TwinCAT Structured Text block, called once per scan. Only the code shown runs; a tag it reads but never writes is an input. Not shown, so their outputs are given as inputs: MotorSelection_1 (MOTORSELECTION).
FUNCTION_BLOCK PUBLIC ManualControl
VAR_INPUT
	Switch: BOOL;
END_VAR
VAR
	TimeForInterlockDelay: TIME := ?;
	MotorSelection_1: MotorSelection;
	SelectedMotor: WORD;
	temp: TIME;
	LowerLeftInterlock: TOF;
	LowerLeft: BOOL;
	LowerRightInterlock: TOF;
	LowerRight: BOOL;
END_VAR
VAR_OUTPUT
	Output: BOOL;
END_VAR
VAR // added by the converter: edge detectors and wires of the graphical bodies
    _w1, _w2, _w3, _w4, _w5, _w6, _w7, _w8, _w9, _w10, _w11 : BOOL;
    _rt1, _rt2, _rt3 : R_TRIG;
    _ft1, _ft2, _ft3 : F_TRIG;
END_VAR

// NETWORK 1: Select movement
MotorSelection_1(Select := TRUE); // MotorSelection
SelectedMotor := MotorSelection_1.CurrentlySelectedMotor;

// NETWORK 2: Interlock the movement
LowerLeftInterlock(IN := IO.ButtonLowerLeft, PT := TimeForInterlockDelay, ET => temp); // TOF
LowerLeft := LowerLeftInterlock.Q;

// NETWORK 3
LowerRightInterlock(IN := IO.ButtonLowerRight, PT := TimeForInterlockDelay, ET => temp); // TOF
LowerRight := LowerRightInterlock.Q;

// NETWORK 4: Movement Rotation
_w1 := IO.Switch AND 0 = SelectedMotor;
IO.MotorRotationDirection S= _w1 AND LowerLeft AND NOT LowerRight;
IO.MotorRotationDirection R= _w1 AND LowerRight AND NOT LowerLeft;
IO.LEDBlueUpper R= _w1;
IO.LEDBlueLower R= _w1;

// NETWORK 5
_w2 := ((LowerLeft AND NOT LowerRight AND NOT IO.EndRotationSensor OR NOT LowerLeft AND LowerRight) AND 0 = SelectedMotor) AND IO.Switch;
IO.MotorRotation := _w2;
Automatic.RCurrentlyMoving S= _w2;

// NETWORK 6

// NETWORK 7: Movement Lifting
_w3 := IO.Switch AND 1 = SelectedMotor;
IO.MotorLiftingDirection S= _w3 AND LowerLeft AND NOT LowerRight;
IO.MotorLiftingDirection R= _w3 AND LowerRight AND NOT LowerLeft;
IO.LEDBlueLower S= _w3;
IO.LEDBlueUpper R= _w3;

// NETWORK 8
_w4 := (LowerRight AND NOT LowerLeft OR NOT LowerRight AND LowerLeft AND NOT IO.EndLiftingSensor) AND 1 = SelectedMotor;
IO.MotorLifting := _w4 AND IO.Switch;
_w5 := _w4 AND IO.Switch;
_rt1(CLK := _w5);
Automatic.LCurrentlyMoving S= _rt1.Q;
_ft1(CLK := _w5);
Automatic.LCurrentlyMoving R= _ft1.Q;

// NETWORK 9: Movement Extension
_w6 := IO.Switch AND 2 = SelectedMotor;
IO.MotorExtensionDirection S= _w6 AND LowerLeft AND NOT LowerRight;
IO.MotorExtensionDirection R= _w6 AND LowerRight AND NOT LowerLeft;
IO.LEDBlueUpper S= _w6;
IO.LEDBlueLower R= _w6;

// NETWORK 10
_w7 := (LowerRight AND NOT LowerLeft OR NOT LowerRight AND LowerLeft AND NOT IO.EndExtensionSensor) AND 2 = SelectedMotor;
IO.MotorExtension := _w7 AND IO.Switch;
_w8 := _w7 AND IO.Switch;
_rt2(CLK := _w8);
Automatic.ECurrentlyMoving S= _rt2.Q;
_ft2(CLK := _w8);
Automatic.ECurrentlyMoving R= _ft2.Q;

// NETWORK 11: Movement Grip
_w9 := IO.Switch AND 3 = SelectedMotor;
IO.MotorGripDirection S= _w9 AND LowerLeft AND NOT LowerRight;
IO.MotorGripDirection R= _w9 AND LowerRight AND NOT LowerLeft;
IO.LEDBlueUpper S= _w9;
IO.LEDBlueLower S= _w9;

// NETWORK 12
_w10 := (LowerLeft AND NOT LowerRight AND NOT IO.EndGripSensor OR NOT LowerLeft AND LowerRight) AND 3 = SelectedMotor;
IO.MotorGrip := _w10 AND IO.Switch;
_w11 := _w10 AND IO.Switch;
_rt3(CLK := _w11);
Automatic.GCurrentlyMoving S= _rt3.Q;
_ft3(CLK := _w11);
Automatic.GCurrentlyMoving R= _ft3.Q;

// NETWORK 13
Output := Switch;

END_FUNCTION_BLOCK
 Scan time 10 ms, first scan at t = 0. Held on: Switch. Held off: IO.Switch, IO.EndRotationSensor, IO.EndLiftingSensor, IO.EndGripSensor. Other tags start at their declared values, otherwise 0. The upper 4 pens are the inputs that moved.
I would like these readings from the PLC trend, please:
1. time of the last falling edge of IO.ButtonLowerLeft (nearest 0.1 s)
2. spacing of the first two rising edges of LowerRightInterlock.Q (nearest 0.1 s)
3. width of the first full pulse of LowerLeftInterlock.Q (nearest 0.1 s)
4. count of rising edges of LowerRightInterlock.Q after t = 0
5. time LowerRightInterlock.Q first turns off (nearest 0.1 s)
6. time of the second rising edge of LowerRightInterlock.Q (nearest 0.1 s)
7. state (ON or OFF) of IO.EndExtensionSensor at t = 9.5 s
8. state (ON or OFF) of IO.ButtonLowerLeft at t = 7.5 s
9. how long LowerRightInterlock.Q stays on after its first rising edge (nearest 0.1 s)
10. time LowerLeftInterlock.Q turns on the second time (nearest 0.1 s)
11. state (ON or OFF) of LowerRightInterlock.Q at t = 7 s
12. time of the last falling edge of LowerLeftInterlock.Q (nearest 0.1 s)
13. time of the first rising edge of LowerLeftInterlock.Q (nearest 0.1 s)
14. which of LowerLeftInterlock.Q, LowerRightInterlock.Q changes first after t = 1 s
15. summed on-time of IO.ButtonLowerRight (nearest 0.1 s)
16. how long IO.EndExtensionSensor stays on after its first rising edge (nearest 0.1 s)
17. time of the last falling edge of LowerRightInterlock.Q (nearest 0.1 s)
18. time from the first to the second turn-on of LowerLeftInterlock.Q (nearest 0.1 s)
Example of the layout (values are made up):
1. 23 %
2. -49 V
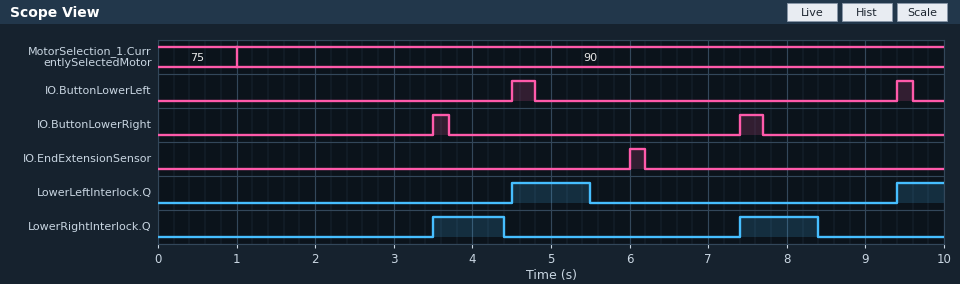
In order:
1. 9.6 s
2. 3.9 s
3. 1.0 s
4. 2
5. 4.4 s
6. 7.4 s
7. OFF
8. OFF
9. 0.9 s
10. 9.4 s
11. OFF
12. 5.5 s
13. 4.5 s
14. LowerRightInterlock.Q
15. 0.5 s
16. 0.2 s
17. 8.4 s
18. 4.9 s
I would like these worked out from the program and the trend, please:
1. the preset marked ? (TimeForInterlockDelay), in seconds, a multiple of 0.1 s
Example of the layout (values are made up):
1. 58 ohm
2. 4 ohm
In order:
1. 0.7 s
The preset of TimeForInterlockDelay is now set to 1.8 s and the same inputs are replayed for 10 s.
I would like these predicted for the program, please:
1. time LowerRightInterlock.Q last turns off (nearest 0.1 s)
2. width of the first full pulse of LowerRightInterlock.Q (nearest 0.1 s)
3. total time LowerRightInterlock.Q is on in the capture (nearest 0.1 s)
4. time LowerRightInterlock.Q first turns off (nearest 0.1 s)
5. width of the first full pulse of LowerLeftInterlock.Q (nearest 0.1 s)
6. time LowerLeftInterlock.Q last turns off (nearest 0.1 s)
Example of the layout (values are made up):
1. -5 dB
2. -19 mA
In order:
1. 9.5 s
2. 2.0 s
3. 4.1 s
4. 5.5 s
5. 2.1 s
6. 6.6 s
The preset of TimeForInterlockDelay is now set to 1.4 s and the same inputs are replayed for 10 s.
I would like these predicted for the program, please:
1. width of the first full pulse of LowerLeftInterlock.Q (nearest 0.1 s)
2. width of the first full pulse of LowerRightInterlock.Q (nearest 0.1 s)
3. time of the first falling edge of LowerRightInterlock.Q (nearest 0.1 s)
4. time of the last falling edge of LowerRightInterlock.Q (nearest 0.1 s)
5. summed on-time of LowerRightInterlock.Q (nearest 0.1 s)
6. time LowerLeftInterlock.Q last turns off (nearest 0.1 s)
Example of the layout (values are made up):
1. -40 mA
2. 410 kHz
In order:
1. 1.7 s
2. 1.6 s
3. 5.1 s
4. 9.1 s
5. 3.3 s
6. 6.2 s
